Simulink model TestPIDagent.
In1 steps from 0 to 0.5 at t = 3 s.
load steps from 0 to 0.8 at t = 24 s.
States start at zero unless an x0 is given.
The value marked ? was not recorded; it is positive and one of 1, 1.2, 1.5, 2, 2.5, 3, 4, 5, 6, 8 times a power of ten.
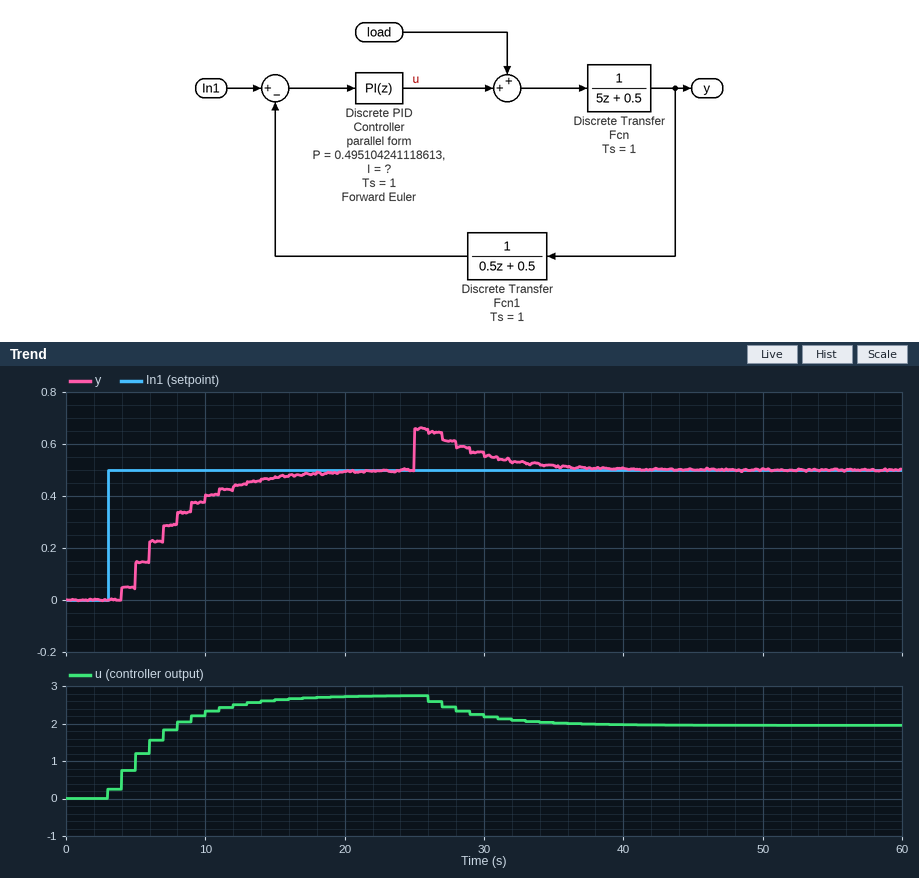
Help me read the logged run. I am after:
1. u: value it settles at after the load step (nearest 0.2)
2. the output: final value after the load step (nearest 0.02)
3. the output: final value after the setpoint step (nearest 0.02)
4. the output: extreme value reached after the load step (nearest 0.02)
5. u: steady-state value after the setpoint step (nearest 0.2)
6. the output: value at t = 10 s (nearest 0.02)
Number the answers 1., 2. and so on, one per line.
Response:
1. 2.0
2. 0.50
3. 0.50
4. 0.66
5. 2.8
6. 0.40
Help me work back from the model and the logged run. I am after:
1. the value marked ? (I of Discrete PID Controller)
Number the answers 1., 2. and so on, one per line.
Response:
1. 1
